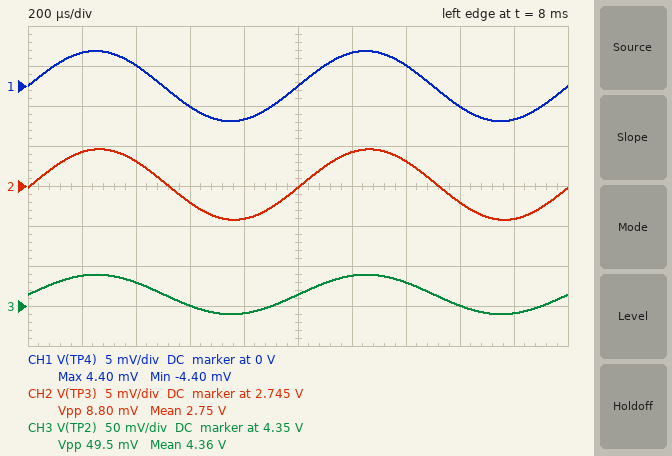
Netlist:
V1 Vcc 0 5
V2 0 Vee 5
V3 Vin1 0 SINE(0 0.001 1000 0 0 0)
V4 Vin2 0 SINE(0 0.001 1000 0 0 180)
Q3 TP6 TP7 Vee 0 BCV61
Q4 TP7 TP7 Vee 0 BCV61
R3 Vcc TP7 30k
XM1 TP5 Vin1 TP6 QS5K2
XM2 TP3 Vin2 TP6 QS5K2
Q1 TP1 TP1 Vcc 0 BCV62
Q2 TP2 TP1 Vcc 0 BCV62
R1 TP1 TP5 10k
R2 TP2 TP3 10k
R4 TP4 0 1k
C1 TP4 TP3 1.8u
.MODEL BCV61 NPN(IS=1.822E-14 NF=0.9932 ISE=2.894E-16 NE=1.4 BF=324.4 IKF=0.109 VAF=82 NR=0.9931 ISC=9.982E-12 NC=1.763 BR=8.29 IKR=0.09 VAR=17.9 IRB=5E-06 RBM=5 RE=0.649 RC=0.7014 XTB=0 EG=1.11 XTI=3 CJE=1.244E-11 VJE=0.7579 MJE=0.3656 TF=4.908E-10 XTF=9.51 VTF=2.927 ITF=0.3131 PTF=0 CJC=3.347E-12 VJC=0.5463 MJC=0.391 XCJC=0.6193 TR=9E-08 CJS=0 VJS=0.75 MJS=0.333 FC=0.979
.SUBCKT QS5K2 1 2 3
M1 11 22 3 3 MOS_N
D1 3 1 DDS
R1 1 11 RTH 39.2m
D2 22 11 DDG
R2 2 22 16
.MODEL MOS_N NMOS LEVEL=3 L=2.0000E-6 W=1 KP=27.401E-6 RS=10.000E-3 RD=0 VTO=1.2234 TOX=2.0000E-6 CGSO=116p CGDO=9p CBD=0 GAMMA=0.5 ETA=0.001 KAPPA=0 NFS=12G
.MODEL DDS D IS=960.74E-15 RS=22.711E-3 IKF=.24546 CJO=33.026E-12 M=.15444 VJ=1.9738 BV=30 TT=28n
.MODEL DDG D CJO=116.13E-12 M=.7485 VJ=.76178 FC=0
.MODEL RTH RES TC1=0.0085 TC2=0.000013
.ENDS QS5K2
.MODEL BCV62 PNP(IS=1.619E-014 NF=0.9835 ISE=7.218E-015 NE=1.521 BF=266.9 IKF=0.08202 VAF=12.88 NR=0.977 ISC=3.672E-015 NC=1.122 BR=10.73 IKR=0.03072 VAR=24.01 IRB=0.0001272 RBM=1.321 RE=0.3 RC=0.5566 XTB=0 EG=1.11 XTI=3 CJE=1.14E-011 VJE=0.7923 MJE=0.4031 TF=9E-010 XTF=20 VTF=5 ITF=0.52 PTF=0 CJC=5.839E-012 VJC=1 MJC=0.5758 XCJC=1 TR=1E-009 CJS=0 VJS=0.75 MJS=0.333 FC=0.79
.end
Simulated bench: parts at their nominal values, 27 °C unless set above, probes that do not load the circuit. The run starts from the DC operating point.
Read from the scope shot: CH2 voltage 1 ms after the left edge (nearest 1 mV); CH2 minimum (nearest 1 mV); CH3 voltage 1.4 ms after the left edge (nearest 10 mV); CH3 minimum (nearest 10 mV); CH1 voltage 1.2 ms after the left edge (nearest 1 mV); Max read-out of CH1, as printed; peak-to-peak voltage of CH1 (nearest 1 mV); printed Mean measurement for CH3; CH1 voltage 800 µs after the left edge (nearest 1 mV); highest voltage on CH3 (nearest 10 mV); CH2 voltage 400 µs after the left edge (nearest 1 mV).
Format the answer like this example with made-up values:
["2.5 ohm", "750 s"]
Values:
["2.745 V", "2.741 V", "4.38 V", "4.34 V", "4 mV", "4.40 mV", "9 mV", "4.36 V", "-4 mV", "4.39 V", "2.748 V"]
